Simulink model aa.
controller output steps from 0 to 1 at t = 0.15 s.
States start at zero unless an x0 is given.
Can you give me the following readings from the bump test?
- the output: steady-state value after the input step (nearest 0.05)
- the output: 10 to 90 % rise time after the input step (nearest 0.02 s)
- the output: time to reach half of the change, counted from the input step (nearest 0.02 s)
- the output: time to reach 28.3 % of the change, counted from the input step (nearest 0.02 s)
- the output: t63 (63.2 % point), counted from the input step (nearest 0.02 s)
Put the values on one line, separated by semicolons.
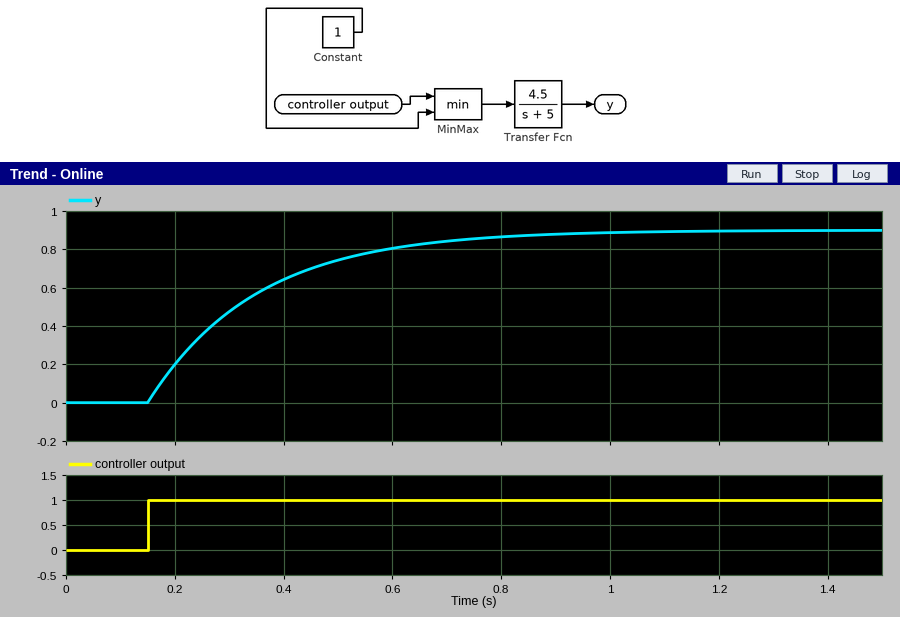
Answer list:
0.90; 0.44 s; 0.14 s; 0.06 s; 0.20 s
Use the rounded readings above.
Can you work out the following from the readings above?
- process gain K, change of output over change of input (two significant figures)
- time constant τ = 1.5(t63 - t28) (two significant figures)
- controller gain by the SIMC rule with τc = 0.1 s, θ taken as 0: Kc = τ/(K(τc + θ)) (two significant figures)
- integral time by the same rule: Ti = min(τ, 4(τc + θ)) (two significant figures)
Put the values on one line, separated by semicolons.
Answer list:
0.90; 0.21 s; 2.3; 0.21 s
